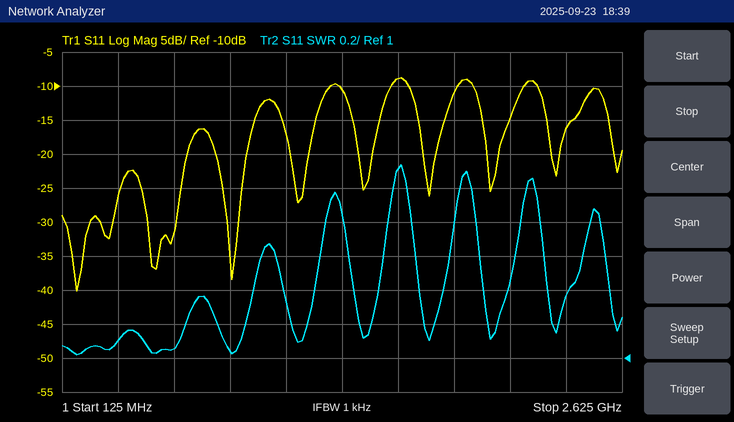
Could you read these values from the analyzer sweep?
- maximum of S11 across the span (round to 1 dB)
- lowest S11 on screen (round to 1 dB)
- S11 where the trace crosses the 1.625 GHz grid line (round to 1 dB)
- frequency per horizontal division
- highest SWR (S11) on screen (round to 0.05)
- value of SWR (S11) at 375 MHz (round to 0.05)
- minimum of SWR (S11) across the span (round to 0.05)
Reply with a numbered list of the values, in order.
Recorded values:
1. -9 dB
2. -40 dB
3. -9 dB
4. 250 MHz
5. 2.15
6. 1.10
7. 1.00
